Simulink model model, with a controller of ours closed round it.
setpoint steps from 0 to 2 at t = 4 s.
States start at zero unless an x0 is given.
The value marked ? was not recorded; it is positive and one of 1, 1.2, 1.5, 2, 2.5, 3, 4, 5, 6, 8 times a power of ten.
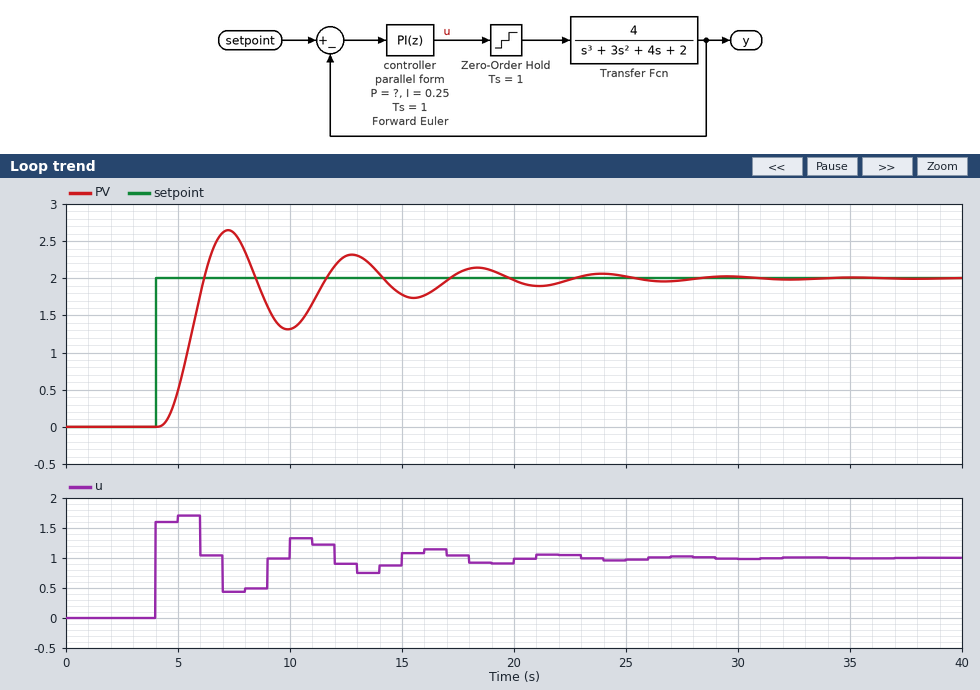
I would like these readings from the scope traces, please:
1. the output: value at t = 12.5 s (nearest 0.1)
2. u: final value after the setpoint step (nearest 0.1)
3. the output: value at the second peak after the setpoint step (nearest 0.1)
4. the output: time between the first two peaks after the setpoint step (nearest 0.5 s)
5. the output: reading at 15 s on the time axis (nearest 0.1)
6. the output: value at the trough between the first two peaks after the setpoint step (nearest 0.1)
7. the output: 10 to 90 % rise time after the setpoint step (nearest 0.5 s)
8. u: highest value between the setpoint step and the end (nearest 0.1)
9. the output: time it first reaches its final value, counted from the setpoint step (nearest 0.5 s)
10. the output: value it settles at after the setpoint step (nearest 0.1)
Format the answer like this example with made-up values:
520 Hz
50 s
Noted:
2.3
1.0
2.3
5.5 s
1.8
1.3
1.5 s
1.7
2.0 s
2.0
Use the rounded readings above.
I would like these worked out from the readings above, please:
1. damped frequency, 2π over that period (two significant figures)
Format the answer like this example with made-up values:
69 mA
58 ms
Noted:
1.1 rad/s
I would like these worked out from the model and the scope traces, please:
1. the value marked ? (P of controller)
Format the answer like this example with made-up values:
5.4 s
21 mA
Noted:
0.8
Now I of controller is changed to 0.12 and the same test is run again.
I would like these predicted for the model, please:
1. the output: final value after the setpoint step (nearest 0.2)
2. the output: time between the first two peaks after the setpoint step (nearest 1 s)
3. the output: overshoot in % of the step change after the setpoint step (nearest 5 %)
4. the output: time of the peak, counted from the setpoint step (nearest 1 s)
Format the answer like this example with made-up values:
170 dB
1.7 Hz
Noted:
2.0
5 s
15 %
3 s
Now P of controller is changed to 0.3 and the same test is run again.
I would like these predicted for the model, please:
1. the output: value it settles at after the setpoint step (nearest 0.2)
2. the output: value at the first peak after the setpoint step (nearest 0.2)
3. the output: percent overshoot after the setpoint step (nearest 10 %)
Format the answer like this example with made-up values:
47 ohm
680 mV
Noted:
2.0
2.6
30 %
